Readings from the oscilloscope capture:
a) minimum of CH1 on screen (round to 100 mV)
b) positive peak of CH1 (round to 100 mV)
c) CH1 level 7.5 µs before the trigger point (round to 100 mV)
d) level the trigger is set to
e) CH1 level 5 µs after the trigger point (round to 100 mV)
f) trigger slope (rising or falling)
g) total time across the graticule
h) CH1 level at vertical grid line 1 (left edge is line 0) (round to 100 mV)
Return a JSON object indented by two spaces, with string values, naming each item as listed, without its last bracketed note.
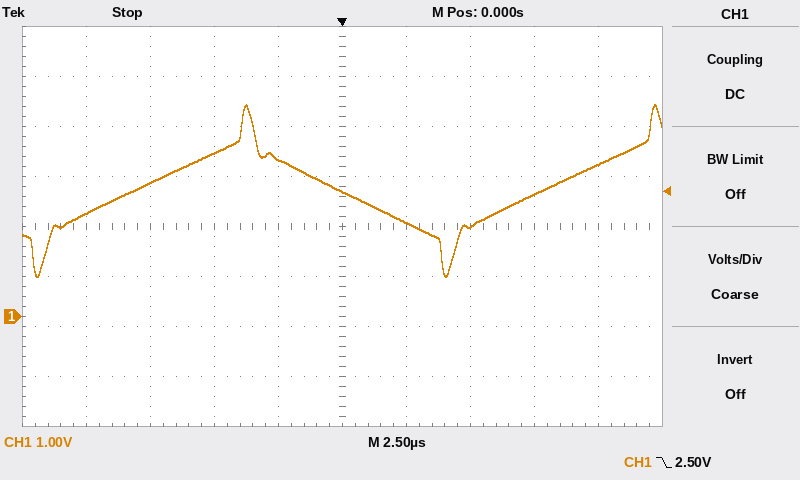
{
  "minimum of CH1 on screen": "800 mV",
  "positive peak of CH1": "4.2 V",
  "CH1 level 7.5 µs before the trigger point": "2.7 V",
  "level the trigger is set to": "2.50 V",
  "CH1 level 5 µs after the trigger point": "1.8 V",
  "trigger slope": "falling",
  "total time across the graticule": "25 µs",
  "CH1 level at vertical grid line 1 (left edge is line 0)": "2.1 V"
}
